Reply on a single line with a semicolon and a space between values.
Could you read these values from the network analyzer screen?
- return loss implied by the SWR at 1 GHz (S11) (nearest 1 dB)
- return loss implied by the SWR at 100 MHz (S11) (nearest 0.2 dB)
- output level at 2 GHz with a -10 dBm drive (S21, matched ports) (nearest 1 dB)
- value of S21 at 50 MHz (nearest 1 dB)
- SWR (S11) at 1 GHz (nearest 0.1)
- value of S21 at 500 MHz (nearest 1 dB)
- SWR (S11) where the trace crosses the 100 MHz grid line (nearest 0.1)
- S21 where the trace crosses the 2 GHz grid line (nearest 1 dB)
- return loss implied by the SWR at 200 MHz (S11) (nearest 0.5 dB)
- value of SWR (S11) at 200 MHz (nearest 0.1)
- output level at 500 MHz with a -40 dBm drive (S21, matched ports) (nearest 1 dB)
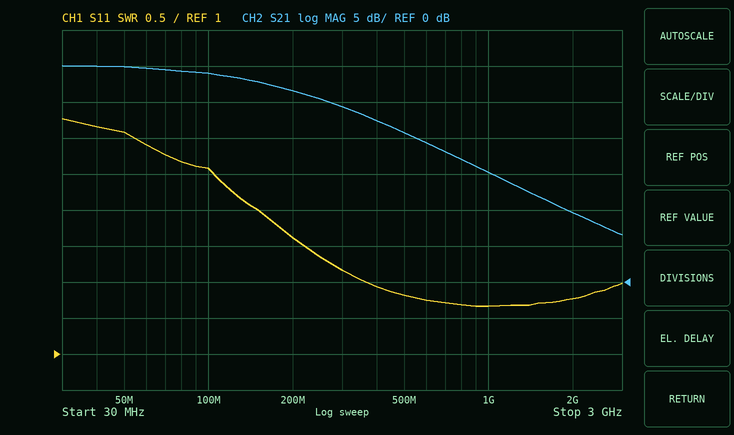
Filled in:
12 dB; 5.0 dB; 0 dBm; 30 dB; 1.7; 21 dB; 3.6; 10 dB; 7.0 dB; 2.6; -19 dBm
